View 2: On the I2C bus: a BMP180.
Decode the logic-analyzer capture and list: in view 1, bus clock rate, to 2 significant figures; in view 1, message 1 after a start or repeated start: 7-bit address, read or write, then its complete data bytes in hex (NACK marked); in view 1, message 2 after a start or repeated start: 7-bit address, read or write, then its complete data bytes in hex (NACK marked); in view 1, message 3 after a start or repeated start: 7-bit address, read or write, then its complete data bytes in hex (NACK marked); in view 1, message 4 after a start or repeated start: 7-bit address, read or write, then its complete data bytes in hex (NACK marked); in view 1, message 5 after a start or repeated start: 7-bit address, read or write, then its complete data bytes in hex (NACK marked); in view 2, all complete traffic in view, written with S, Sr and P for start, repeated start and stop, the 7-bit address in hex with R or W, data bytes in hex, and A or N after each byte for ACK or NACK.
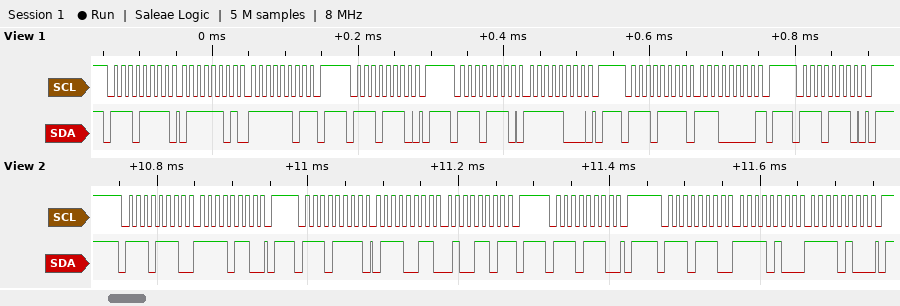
100 kHz
0x77 read: 7D FD NACK
0x77 write
0x77 write: F8
0x77 read: E0 NACK
0x77 write
S 77W A F6 A P S 77R A 73 A 4D N P S 77W A P S 77W A F4 A F4 A P
